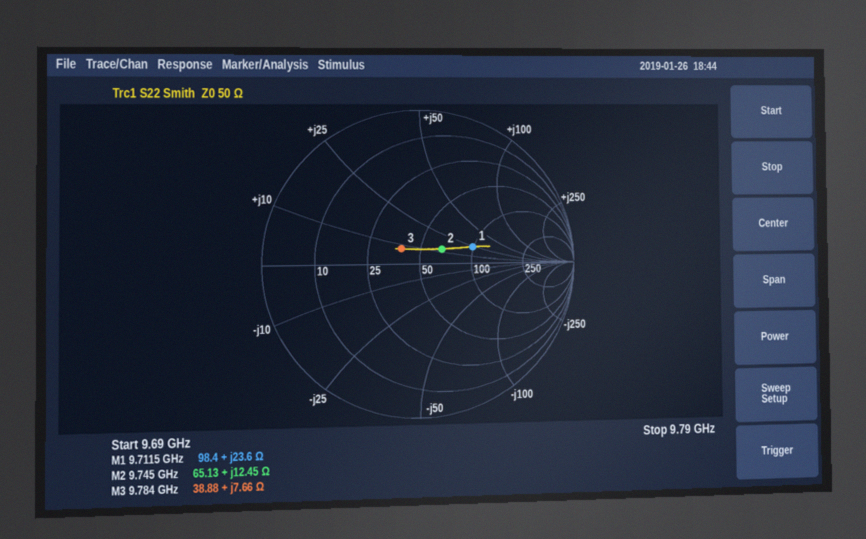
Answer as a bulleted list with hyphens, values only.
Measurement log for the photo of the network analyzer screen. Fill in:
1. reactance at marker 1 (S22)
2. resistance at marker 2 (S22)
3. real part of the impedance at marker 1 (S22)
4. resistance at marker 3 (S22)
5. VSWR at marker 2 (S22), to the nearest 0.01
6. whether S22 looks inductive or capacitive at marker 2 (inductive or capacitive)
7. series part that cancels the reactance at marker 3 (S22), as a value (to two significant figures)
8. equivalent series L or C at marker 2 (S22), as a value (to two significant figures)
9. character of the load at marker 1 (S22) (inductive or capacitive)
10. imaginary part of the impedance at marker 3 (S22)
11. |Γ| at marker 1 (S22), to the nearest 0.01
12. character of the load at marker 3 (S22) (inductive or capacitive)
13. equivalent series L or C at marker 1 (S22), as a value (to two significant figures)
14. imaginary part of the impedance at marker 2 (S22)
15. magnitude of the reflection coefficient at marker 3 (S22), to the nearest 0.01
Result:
- +23.6 Ω
- 65.13 Ω
- 98.4 Ω
- 38.88 Ω
- 1.41
- inductive
- 2.1 pF
- 200 pH
- inductive
- +7.66 Ω
- 0.36
- inductive
- 390 pH
- +12.45 Ω
- 0.15
